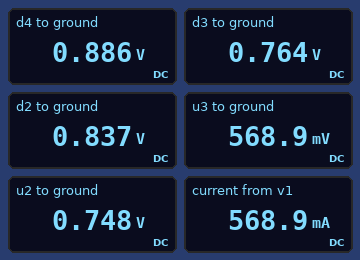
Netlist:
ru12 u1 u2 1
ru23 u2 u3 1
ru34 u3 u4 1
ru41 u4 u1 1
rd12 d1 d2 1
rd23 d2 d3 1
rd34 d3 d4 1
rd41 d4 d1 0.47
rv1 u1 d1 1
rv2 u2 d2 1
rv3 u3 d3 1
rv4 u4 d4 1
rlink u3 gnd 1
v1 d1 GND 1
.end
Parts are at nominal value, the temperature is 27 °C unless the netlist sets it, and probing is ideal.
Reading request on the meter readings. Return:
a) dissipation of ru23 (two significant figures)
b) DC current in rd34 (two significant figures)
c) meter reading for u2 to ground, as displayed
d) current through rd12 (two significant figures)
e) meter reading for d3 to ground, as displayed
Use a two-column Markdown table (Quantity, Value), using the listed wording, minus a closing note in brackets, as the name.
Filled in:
| Quantity | Value |
|---|---|
| dissipation of ru23 | 32 mW |
| DC current in rd34 | 120 mA |
| meter reading for u2 to ground, as displayed | 0.748 V |
| current through rd12 | 160 mA |
| meter reading for d3 to ground, as displayed | 0.764 V |
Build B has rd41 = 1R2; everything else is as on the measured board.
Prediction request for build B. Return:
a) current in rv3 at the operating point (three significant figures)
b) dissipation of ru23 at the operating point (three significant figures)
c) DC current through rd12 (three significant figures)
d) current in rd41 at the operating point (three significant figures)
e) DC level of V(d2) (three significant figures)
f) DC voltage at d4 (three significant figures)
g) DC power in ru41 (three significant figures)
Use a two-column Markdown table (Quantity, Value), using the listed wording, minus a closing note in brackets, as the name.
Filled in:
| Quantity | Value |
|---|---|
| current in rv3 at the operating point | 178 mA |
| dissipation of ru23 at the operating point | 33.3 mW |
| DC current through rd12 | 187 mA |
| current in rd41 at the operating point | 166 mA |
| DC level of V(d2) | 813 mV |
| DC voltage at d4 | 801 mV |
| DC power in ru41 | 9.11 mW |
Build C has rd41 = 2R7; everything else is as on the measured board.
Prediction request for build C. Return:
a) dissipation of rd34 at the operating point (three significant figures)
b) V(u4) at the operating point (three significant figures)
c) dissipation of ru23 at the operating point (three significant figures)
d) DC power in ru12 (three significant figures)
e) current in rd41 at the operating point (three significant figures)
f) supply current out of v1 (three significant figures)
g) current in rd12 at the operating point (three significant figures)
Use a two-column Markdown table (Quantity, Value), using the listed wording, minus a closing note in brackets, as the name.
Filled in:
| Quantity | Value |
|---|---|
| dissipation of rd34 at the operating point | 2.52 mW |
| V(u4) at the operating point | 679 mV |
| dissipation of ru23 at the operating point | 34.5 mW |
| DC power in ru12 | 8.62 mW |
| current in rd41 at the operating point | 100 mA |
| supply current out of v1 | 514 mA |
| current in rd12 at the operating point | 207 mA |
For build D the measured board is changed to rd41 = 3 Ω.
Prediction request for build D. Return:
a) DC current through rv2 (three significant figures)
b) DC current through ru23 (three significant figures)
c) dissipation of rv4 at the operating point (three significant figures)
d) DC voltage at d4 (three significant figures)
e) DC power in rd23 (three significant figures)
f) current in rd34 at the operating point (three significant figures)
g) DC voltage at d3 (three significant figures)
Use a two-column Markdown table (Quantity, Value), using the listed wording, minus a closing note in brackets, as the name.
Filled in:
| Quantity | Value |
|---|---|
| DC current through rv2 | 93.0 mA |
| DC current through ru23 | 186 mA |
| dissipation of rv4 at the operating point | 2.16 mW |
| DC voltage at d4 | 721 mV |
| DC power in rd23 | 13.5 mW |
| current in rd34 at the operating point | 46.5 mA |
| DC voltage at d3 | 674 mV |
